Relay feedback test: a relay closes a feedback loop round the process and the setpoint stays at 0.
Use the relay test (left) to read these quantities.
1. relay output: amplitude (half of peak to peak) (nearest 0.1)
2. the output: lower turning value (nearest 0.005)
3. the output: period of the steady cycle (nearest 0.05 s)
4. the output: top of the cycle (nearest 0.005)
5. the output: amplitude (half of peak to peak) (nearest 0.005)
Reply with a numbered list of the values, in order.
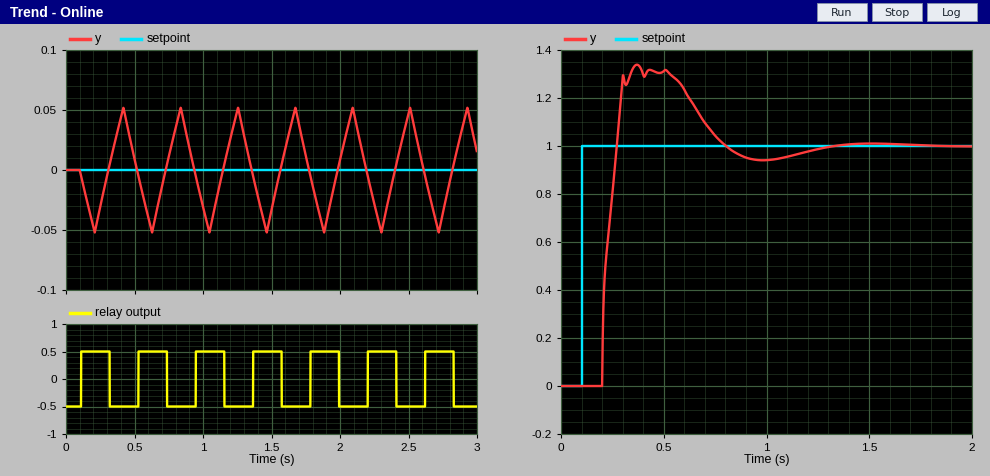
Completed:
1. 0.5
2. -0.050
3. 0.40 s
4. 0.050
5. 0.050
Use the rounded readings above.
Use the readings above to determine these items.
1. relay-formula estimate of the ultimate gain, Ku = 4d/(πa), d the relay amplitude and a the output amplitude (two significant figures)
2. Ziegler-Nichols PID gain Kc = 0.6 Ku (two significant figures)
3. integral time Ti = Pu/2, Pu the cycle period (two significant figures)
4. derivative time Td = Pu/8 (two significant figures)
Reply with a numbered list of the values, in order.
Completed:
1. 13
2. 7.8
3. 0.20 s
4. 0.050 s
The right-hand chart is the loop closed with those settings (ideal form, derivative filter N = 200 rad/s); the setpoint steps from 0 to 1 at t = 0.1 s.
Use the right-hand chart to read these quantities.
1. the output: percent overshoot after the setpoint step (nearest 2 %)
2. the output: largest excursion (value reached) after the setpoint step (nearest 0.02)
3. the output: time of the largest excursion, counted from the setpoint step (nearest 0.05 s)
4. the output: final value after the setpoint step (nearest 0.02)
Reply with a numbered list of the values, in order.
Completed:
1. 34 %
2. 1.34
3. 0.25 s
4. 1.00
